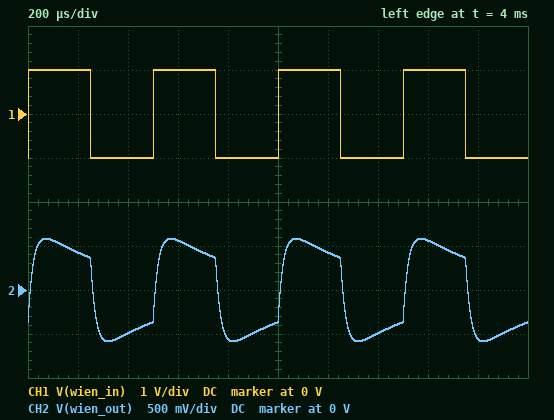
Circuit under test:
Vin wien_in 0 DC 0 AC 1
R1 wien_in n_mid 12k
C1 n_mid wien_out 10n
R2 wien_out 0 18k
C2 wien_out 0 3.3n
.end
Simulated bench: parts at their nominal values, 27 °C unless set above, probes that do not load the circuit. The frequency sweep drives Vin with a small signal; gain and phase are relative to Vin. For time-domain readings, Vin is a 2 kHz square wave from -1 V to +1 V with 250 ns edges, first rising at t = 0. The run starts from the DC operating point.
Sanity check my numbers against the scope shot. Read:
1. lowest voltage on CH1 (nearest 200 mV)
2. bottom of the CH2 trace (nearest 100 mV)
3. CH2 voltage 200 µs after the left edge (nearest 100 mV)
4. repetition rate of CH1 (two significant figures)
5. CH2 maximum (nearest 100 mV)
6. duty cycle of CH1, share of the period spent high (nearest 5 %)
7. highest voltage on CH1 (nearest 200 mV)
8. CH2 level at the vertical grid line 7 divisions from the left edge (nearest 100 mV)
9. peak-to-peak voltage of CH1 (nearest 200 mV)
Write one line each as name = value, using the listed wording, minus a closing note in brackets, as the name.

lowest voltage on CH1 = -1.0 V
bottom of the CH2 trace = -600 mV
CH2 voltage 200 µs after the left edge = 400 mV
repetition rate of CH1 = 2.0 kHz
CH2 maximum = 600 mV
duty cycle of CH1, share of the period spent high = 50 %
highest voltage on CH1 = 1.0 V
CH2 level at the vertical grid line 7 divisions from the left edge = -500 mV
peak-to-peak voltage of CH1 = 2.0 V
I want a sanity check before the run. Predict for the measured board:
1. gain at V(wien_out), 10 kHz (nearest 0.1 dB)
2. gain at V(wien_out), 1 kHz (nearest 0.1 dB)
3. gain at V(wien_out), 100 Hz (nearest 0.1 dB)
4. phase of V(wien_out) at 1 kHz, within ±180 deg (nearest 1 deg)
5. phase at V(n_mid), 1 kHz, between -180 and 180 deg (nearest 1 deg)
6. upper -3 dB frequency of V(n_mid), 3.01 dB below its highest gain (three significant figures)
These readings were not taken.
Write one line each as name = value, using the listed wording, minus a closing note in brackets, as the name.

gain at V(wien_out), 10 kHz = -9.9 dB
gain at V(wien_out), 1 kHz = -6.4 dB
gain at V(wien_out), 100 Hz = -19.1 dB
phase of V(wien_out) at 1 kHz, within ±180 deg = 18 deg
phase at V(n_mid), 1 kHz, between -180 and 180 deg = -16 deg
upper -3 dB frequency of V(n_mid), 3.01 dB below its highest gain = 1.87 kHz
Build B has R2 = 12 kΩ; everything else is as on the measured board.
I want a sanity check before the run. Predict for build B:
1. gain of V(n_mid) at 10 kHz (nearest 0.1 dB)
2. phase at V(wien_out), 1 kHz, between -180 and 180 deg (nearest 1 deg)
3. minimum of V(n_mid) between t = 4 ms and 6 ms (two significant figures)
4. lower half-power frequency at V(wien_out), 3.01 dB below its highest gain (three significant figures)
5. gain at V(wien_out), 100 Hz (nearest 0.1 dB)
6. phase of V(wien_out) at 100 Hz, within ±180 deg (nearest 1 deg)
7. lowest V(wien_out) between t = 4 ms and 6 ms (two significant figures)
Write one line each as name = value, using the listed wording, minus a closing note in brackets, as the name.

gain of V(n_mid) at 10 kHz = -7.9 dB
phase at V(wien_out), 1 kHz, between -180 and 180 deg = 25 deg
minimum of V(n_mid) between t = 4 ms and 6 ms = -770 mV
lower half-power frequency at V(wien_out), 3.01 dB below its highest gain = 538 Hz
gain at V(wien_out), 100 Hz = -22.6 dB
phase of V(wien_out) at 100 Hz, within ±180 deg = 80 deg
lowest V(wien_out) between t = 4 ms and 6 ms = -530 mV
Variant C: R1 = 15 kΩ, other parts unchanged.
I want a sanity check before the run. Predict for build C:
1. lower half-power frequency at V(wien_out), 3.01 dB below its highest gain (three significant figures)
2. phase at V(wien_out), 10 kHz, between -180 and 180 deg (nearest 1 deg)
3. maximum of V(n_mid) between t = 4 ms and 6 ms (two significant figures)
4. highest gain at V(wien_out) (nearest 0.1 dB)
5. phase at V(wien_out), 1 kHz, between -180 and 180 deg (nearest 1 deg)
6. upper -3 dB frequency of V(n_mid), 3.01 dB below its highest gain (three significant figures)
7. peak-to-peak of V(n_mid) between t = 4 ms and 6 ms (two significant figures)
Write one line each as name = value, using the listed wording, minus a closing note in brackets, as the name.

lower half-power frequency at V(wien_out), 3.01 dB below its highest gain = 387 Hz
phase at V(wien_out), 10 kHz, between -180 and 180 deg = -54 deg
maximum of V(n_mid) between t = 4 ms and 6 ms = 750 mV
highest gain at V(wien_out) = -6.7 dB
phase at V(wien_out), 1 kHz, between -180 and 180 deg = 15 deg
upper -3 dB frequency of V(n_mid), 3.01 dB below its highest gain = 1.06 kHz
peak-to-peak of V(n_mid) between t = 4 ms and 6 ms = 1.5 V
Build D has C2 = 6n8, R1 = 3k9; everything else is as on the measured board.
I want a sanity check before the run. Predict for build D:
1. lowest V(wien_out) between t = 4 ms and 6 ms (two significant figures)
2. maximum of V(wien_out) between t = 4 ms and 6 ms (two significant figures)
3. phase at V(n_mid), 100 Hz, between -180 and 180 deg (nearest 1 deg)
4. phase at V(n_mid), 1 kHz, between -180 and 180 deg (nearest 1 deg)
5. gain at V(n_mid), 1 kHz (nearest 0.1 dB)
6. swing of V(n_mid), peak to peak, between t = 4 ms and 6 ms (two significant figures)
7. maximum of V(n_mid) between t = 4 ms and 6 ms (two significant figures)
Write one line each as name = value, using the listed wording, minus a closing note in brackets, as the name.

lowest V(wien_out) between t = 4 ms and 6 ms = -640 mV
maximum of V(wien_out) between t = 4 ms and 6 ms = 640 mV
phase at V(n_mid), 100 Hz, between -180 and 180 deg = -1 deg
phase at V(n_mid), 1 kHz, between -180 and 180 deg = -7 deg
gain at V(n_mid), 1 kHz = -0.6 dB
swing of V(n_mid), peak to peak, between t = 4 ms and 6 ms = 1.9 V
maximum of V(n_mid) between t = 4 ms and 6 ms = 950 mV
